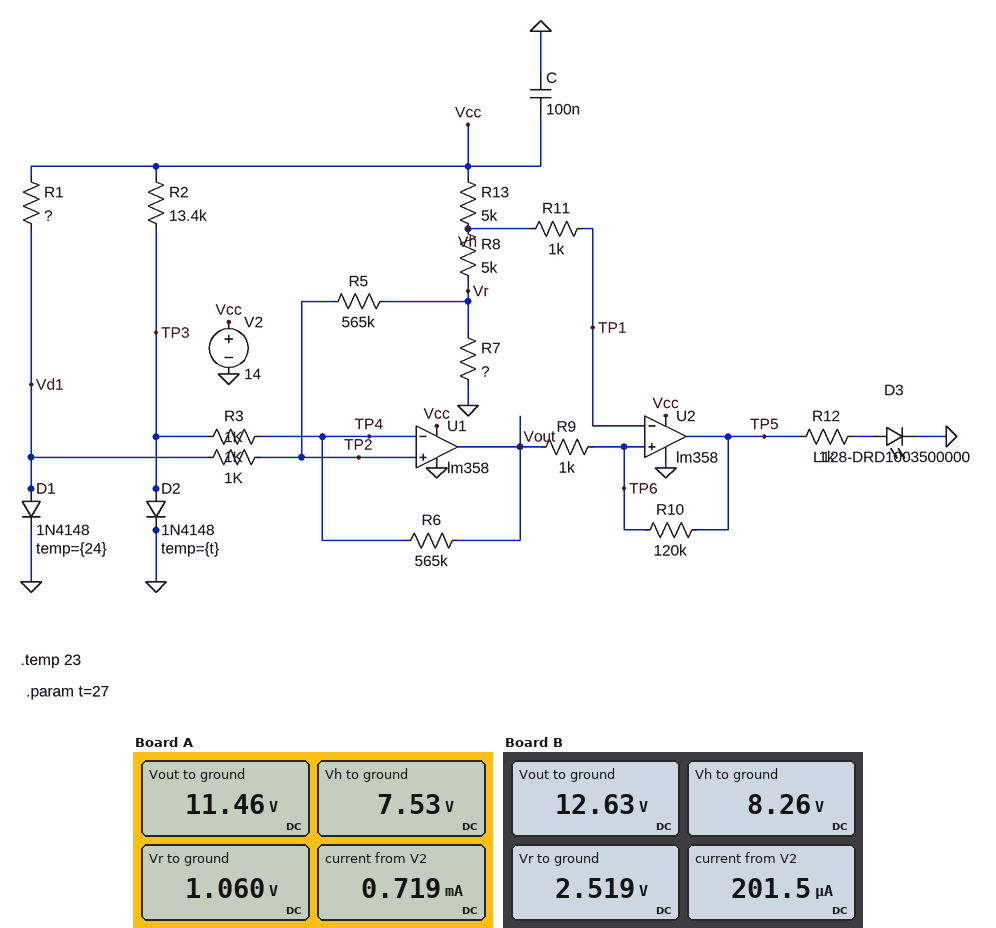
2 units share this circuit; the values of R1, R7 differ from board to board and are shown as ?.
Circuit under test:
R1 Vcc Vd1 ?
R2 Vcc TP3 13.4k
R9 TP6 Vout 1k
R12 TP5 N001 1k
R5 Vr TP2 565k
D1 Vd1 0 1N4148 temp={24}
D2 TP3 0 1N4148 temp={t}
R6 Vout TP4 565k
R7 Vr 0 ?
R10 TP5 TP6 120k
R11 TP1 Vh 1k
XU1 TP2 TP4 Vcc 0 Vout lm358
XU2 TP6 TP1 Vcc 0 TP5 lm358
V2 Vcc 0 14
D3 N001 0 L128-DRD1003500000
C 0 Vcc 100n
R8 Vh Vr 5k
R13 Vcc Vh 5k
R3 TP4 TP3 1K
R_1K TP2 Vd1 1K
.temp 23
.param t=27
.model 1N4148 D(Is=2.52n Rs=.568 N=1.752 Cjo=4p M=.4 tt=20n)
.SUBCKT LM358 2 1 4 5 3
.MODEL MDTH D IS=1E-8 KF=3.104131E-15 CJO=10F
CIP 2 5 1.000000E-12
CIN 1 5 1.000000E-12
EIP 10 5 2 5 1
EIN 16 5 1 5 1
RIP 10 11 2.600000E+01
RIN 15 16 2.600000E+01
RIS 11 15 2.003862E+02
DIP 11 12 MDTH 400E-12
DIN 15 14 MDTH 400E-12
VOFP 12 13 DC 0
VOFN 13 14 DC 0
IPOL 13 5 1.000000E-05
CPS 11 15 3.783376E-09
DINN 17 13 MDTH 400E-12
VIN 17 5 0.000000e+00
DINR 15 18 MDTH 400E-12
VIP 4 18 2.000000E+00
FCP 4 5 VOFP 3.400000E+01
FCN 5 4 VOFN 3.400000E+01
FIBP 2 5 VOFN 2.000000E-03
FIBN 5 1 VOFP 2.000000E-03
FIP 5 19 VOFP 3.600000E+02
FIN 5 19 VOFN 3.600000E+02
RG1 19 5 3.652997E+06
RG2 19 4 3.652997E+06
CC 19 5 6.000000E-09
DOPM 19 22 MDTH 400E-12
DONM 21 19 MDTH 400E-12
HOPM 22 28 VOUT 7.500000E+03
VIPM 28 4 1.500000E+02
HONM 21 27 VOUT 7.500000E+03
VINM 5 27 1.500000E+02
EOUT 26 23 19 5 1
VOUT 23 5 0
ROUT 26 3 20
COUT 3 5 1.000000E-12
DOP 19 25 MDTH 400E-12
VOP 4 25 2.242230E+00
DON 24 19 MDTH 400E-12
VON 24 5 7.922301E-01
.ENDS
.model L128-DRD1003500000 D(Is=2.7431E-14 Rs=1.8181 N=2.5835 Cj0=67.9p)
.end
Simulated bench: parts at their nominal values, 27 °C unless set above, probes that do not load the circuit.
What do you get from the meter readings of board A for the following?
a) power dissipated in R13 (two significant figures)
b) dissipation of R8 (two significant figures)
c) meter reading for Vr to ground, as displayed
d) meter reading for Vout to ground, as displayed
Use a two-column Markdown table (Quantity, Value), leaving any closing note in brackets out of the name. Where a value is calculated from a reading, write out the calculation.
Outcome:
| Quantity | Value |
|---|---|
| power dissipated in R13 | (14 V - 7.53 V)^2 / 5 kΩ = 8.4 mW |
| dissipation of R8 | (7.53 V - 1.06 V)^2 / 5 kΩ = 8.4 mW |
| meter reading for Vr to ground, as displayed | 1.060 V |
| meter reading for Vout to ground, as displayed | 11.46 V |
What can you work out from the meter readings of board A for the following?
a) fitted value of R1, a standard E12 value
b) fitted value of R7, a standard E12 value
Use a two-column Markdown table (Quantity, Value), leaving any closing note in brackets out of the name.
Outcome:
| Quantity | Value |
|---|---|
| fitted value of R1, a standard E12 value | 10 kΩ |
| fitted value of R7, a standard E12 value | 820 Ω |
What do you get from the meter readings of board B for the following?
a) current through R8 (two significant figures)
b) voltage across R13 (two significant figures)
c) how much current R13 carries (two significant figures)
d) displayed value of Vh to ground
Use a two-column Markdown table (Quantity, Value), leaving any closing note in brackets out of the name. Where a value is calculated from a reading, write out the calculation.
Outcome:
| Quantity | Value |
|---|---|
| current through R8 | (8.26 V - 2.519 V) / 5 kΩ = 1.1 mA |
| voltage across R13 | 14 V - 8.26 V = 5.7 V |
| how much current R13 carries | (14 V - 8.26 V) / 5 kΩ = 1.1 mA |
| displayed value of Vh to ground | 8.26 V |
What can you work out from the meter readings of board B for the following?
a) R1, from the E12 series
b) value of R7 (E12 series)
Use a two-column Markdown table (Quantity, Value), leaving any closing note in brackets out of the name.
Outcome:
| Quantity | Value |
|---|---|
| R1, from the E12 series | 5.6 kΩ |
| value of R7 | 2.2 kΩ |
